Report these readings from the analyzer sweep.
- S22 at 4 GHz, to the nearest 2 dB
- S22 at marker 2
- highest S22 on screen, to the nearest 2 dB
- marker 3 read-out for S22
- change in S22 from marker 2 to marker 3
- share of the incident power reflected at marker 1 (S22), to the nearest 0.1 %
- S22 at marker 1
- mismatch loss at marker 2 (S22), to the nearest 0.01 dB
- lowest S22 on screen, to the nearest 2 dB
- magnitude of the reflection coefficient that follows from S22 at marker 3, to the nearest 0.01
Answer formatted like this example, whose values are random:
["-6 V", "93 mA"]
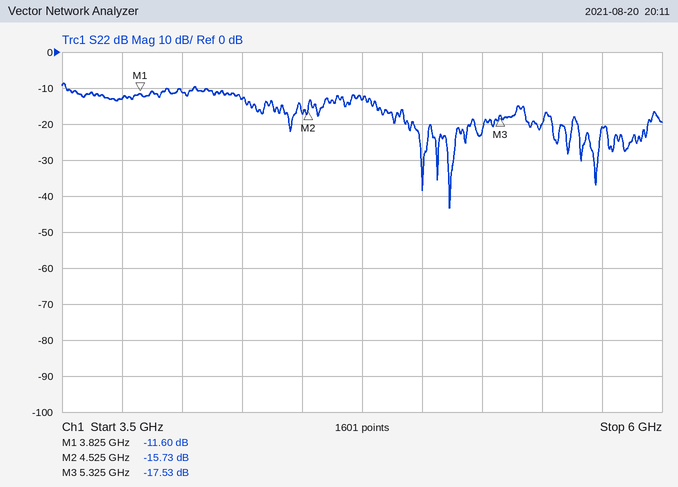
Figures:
["-12 dB", "-15.73 dB", "-8 dB", "-17.53 dB", "-1.80 dB", "6.9 %", "-11.60 dB", "0.12 dB", "-44 dB", "0.13"]
